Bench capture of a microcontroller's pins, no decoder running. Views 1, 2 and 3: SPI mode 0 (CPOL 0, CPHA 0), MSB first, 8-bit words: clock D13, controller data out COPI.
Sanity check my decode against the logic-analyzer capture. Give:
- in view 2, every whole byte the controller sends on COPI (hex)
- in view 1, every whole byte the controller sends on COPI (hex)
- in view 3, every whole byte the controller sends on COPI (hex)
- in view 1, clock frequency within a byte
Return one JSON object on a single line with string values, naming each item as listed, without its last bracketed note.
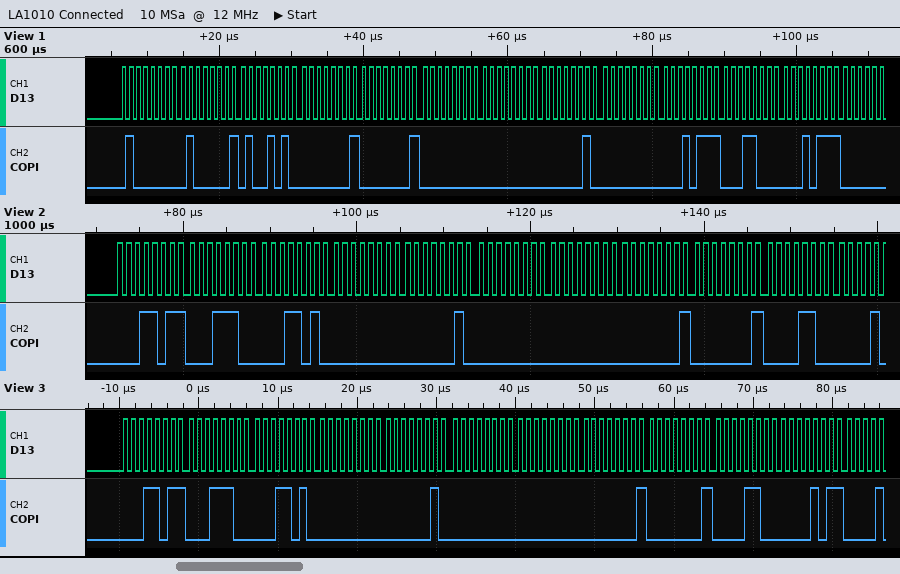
{"in view 2, every whole byte the controller sends on COPI": "1B 1C 1A 00 02 00 00 01 01 0C", "in view 1, every whole byte the controller sends on COPI": "40 41 4A 01 01 00 00 02 00 17 18 17", "in view 3, every whole byte the controller sends on COPI": "0x1B 0x1C 0x1A 0x00 0x02 0x00 0x00 0x01 0x01 0x0C 0x0B", "in view 1, clock frequency within a byte": "1 MHz"}
